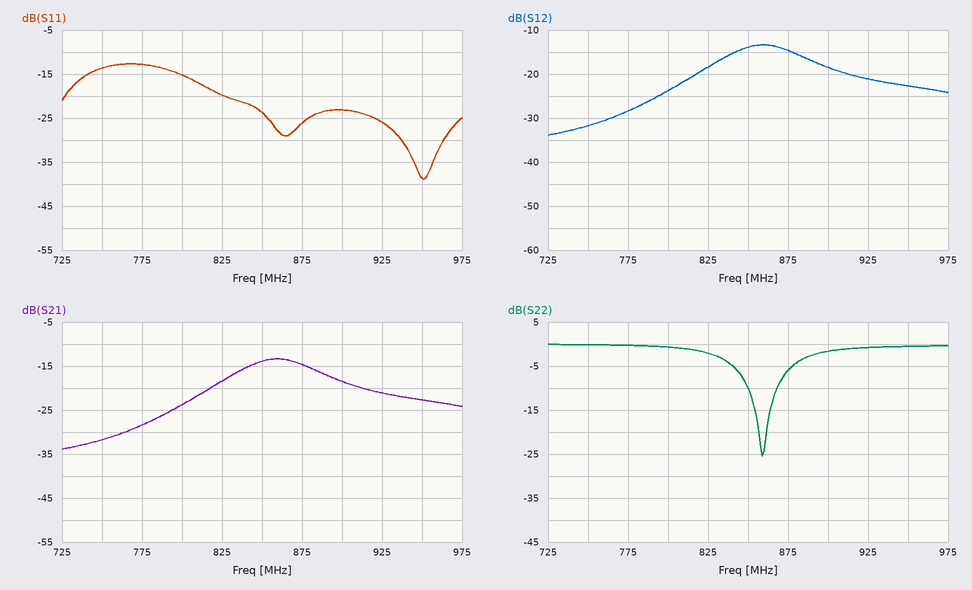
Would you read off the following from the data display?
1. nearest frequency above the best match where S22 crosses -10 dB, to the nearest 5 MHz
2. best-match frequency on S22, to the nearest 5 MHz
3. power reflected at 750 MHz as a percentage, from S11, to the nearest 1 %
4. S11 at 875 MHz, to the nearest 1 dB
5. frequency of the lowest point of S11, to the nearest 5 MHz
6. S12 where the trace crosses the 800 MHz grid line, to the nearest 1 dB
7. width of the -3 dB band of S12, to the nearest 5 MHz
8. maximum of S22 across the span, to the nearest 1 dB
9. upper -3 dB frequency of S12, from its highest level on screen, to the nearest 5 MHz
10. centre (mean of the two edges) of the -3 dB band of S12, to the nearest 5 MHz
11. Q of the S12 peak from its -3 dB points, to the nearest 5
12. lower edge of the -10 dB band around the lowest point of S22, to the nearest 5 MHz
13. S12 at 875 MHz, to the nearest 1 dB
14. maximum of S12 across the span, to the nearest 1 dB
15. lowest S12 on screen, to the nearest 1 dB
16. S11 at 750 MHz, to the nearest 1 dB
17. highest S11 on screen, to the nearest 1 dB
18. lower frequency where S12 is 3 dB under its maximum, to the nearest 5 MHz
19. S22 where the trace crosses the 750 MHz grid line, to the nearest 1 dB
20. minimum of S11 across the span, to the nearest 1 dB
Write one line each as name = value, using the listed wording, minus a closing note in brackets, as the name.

nearest frequency above the best match where S22 crosses -10 dB, to the nearest 5 MHz = 870 MHz
best-match frequency on S22, to the nearest 5 MHz = 860 MHz
power reflected at 750 MHz as a percentage, from S11, to the nearest 1 % = 4 %
S11 at 875 MHz, to the nearest 1 dB = -26 dB
frequency of the lowest point of S11, to the nearest 5 MHz = 950 MHz
S12 where the trace crosses the 800 MHz grid line, to the nearest 1 dB = -24 dB
width of the -3 dB band of S12, to the nearest 5 MHz = 50 MHz
maximum of S22 across the span, to the nearest 1 dB = 0 dB
upper -3 dB frequency of S12, from its highest level on screen, to the nearest 5 MHz = 885 MHz
centre (mean of the two edges) of the -3 dB band of S12, to the nearest 5 MHz = 860 MHz
Q of the S12 peak from its -3 dB points, to the nearest 5 = 15
lower edge of the -10 dB band around the lowest point of S22, to the nearest 5 MHz = 850 MHz
S12 at 875 MHz, to the nearest 1 dB = -15 dB
maximum of S12 across the span, to the nearest 1 dB = -13 dB
lowest S12 on screen, to the nearest 1 dB = -34 dB
S11 at 750 MHz, to the nearest 1 dB = -14 dB
highest S11 on screen, to the nearest 1 dB = -13 dB
lower frequency where S12 is 3 dB under its maximum, to the nearest 5 MHz = 835 MHz
S22 where the trace crosses the 750 MHz grid line, to the nearest 1 dB = 0 dB
minimum of S11 across the span, to the nearest 1 dB = -39 dB
